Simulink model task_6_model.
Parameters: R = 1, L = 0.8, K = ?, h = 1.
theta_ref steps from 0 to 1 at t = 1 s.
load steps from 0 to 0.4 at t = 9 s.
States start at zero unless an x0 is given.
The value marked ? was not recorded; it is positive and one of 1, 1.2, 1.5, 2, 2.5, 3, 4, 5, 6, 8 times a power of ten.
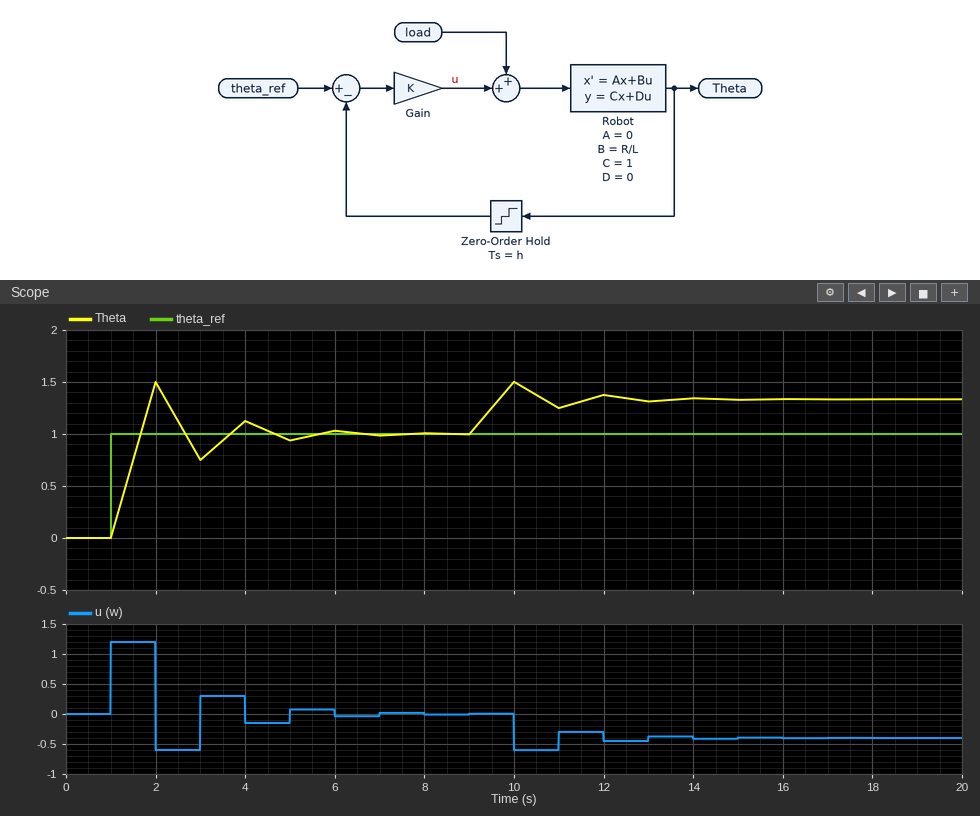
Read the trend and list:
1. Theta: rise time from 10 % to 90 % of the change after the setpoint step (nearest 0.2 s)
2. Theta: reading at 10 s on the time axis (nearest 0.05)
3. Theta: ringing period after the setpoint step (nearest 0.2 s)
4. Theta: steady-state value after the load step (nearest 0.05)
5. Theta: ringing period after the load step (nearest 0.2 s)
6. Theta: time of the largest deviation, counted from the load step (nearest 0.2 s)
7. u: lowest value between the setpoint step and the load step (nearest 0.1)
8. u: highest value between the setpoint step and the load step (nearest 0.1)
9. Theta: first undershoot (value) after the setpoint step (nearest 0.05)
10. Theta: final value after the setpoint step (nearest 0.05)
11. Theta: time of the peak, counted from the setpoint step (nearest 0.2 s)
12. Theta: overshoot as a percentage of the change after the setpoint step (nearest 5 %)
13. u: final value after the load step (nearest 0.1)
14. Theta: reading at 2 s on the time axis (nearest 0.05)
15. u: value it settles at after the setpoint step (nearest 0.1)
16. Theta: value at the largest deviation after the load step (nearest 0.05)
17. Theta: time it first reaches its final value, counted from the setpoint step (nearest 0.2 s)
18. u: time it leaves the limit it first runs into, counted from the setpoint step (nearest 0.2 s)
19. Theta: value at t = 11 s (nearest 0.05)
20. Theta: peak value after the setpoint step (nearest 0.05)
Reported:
0.6 s
1.50
2.0 s
1.35
2.0 s
1.0 s
-0.6
1.2
0.75
1.00
1.0 s
50 %
-0.4
1.50
0.0
1.50
0.6 s
1.0 s
1.25
1.50
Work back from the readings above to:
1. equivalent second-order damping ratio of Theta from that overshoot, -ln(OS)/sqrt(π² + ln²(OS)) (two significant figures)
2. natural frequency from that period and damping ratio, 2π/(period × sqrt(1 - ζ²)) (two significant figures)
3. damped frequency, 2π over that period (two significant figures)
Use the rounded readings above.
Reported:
0.22
3.2 rad/s
3.1 rad/s
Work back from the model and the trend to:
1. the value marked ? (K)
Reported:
1.2
